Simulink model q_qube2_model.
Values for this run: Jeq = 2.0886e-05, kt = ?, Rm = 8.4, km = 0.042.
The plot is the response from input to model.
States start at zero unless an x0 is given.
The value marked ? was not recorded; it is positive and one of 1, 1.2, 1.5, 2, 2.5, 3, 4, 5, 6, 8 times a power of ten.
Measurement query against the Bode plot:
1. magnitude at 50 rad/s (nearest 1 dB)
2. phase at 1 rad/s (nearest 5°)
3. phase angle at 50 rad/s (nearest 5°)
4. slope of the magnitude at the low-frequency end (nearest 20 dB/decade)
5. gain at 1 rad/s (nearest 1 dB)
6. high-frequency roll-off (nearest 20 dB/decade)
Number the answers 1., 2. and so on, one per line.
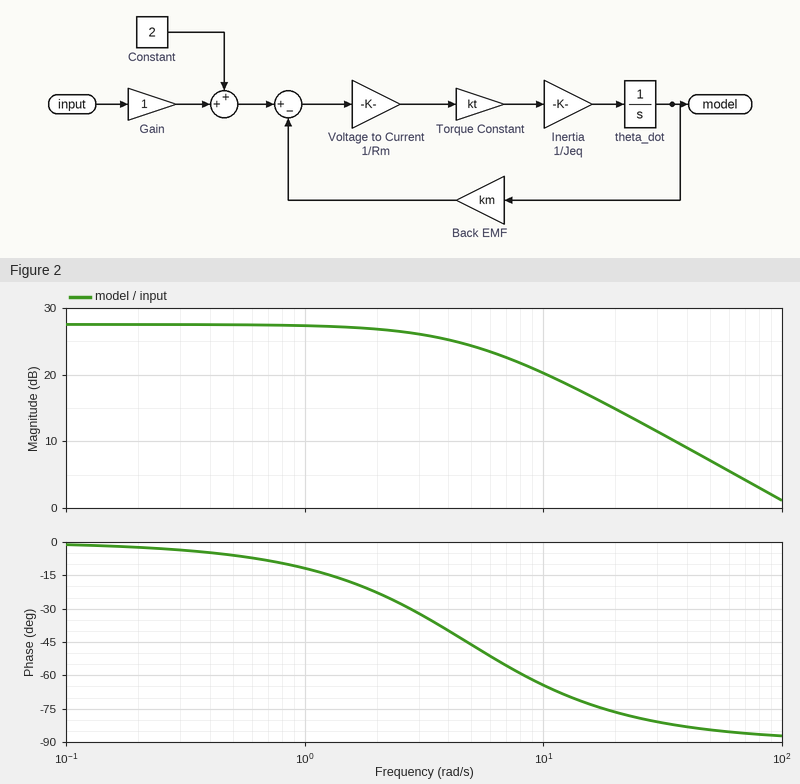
1. 7 dB
2. -10°
3. -85°
4. 0 dB/decade
5. 27 dB
6. -20 dB/decade
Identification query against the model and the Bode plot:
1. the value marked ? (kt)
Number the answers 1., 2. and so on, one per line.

1. 0.02
